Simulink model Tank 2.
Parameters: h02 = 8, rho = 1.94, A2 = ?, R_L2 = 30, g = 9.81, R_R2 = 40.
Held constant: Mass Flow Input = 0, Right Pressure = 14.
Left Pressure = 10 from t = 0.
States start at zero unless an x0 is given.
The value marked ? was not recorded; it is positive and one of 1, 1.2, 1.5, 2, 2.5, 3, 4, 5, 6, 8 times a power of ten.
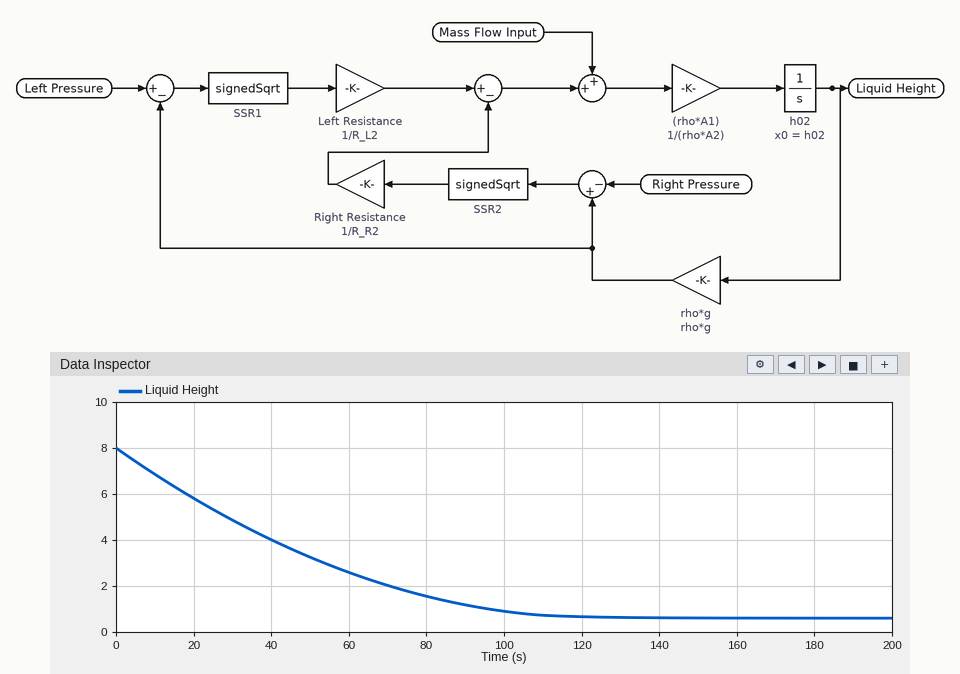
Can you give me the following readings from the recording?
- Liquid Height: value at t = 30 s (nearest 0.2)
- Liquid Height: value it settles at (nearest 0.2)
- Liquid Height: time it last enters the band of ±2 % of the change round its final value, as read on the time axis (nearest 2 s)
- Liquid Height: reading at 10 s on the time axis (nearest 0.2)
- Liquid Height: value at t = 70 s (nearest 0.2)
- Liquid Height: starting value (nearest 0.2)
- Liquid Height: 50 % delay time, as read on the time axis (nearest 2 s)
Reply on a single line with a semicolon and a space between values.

4.8; 0.6; 108 s; 6.8; 2.0; 8.0; 36 s
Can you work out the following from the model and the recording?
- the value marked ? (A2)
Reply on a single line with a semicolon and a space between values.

3
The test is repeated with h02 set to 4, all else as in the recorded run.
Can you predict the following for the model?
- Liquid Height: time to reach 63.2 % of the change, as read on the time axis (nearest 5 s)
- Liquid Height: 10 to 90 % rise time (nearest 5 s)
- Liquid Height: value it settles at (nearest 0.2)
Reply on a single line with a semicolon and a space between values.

35 s; 55 s; 0.6
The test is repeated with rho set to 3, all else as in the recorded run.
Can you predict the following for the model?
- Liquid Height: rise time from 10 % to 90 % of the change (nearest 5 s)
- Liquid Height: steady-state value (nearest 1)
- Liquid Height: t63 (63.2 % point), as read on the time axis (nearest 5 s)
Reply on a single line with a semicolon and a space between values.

100 s; 0; 60 s
